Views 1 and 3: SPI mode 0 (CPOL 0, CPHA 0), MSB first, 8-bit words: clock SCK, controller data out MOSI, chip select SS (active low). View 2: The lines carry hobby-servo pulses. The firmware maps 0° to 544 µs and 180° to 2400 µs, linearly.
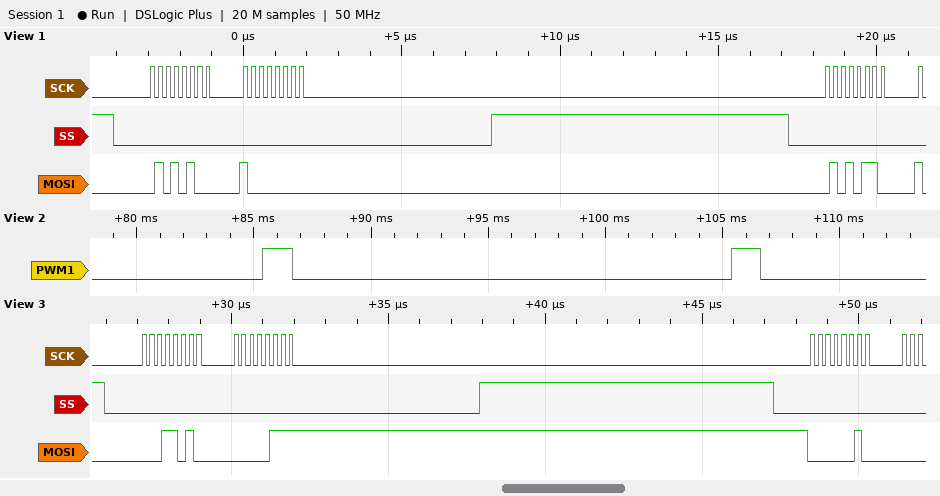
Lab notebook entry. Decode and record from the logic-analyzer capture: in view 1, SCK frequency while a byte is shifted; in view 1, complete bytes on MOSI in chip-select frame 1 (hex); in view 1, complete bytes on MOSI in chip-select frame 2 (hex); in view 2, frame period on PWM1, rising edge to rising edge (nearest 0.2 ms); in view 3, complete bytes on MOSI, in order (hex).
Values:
4 MHz
54 80
56
20.0 ms
1A 07 02
